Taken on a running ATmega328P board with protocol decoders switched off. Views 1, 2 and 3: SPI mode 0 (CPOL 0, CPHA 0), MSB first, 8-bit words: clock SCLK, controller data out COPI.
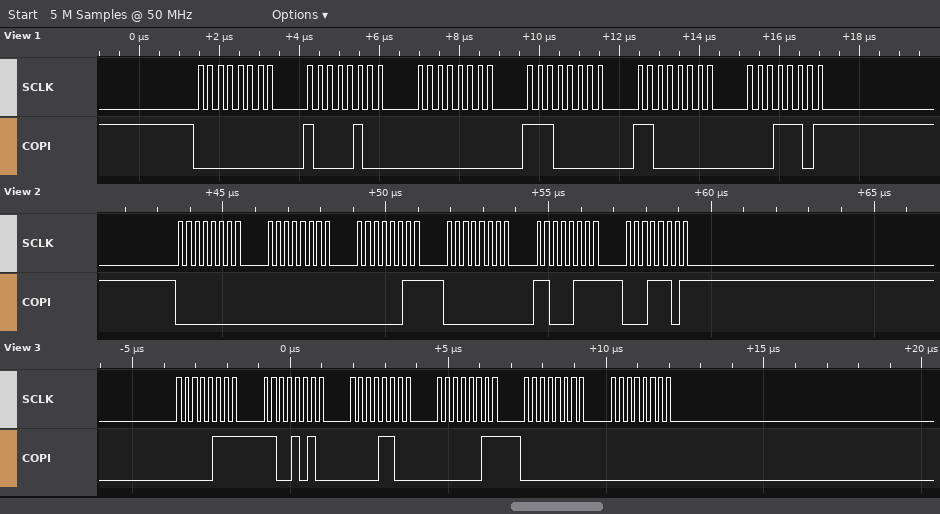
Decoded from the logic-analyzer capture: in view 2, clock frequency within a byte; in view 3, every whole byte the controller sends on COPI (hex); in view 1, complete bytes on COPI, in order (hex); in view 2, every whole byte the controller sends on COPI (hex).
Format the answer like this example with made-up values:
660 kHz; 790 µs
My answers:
4 MHz; 07 CA 0C 03 00 00; 00 84 00 E0 C0 1D; 00 00 03 00 C7 1D
